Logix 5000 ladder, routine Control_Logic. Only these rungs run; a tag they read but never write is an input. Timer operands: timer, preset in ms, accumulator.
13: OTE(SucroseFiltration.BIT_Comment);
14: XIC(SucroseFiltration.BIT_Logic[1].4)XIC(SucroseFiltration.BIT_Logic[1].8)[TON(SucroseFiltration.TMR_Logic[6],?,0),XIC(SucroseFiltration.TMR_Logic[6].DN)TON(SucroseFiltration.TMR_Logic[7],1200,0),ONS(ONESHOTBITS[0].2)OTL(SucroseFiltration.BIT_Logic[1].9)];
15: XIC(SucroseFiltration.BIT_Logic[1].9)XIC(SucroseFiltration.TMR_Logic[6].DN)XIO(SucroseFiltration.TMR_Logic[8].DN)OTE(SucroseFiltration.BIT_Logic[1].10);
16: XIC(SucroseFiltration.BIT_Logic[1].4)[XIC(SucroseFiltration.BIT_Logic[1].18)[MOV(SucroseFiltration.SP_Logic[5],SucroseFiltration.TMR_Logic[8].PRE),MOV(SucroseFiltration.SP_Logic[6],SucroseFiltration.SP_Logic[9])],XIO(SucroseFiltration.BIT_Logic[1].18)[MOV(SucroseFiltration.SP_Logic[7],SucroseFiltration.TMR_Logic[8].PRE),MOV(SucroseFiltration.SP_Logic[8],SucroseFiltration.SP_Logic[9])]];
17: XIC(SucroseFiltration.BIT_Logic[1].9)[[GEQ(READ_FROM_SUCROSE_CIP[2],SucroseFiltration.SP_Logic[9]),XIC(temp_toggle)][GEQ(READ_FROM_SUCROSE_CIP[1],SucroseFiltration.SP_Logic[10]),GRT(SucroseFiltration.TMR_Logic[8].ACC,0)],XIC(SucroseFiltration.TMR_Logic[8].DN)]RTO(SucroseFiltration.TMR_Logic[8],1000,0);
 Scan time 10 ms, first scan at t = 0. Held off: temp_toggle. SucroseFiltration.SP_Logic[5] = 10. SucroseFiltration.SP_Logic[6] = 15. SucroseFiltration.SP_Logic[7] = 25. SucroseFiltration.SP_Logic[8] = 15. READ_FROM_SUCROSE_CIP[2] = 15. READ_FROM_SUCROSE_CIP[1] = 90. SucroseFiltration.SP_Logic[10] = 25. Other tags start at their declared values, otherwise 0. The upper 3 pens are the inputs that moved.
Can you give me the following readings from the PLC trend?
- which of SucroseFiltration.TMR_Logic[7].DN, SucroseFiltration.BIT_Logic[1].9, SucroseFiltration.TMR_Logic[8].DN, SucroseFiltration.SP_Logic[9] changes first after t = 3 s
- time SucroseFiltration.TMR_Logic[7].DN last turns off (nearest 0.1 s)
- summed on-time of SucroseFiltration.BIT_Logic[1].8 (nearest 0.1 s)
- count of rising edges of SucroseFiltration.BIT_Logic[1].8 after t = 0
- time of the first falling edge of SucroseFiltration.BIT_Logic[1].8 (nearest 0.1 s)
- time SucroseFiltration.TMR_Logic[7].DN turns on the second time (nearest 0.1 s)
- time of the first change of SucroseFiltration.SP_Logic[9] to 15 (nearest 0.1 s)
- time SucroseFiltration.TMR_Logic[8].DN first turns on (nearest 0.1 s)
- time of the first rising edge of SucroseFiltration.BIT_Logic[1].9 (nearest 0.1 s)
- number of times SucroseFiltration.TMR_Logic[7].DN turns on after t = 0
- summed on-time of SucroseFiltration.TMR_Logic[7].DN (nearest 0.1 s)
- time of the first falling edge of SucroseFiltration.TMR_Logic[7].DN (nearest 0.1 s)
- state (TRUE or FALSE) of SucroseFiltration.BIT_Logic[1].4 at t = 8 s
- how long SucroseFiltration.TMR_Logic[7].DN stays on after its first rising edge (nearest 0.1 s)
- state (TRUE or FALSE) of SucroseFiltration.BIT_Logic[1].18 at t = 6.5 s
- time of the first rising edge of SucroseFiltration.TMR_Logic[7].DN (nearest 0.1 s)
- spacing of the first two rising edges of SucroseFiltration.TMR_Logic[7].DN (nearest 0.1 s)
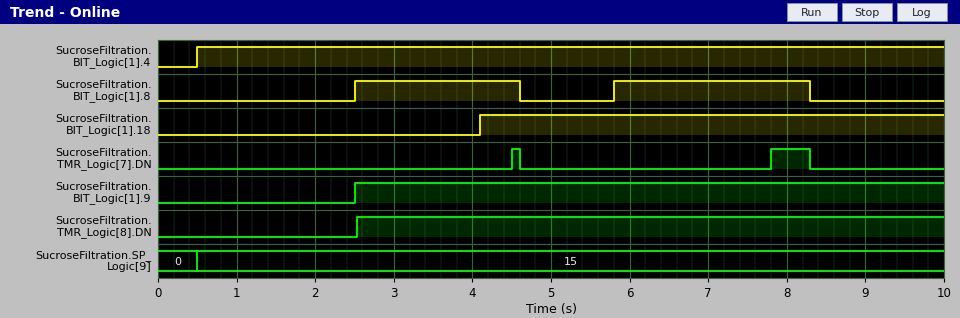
SucroseFiltration.TMR_Logic[7].DN
8.3 s
4.6 s
2
4.6 s
7.8 s
0.5 s
2.5 s
2.5 s
2
0.6 s
4.6 s
TRUE
0.1 s
TRUE
4.5 s
3.3 s
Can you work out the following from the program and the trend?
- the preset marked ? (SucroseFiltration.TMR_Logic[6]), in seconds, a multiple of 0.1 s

0.8 s
